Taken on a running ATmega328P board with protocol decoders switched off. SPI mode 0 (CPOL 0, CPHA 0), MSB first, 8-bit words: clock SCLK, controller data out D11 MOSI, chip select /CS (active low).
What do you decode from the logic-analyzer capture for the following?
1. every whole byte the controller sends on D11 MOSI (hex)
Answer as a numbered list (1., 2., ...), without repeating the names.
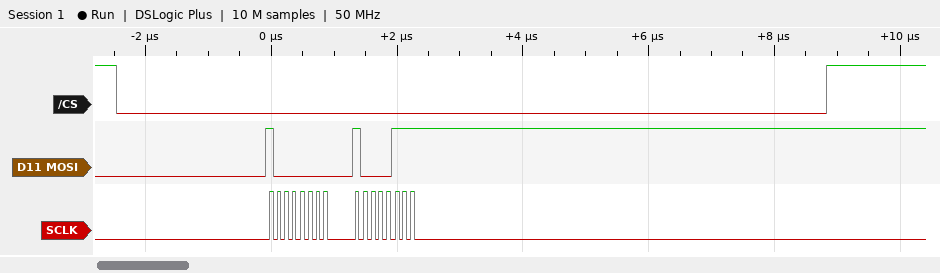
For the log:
1. 0x80 0x87
